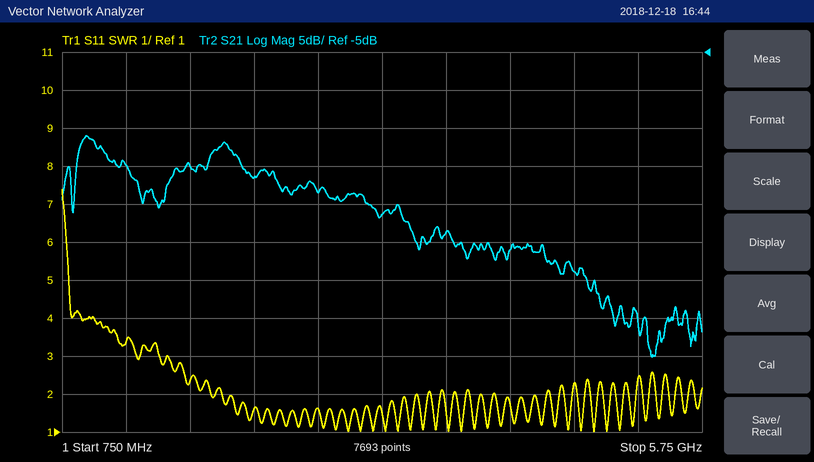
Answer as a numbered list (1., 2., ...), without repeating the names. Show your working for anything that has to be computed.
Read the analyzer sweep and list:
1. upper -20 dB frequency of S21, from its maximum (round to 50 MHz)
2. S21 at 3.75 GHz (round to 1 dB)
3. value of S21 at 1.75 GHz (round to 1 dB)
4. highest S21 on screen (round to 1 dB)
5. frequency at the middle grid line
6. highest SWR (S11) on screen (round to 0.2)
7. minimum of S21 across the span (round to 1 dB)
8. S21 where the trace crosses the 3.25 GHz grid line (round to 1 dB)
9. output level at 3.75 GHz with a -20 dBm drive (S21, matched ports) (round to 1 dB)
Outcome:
1. 4.85 GHz
2. -29 dB
3. -20 dB
4. -16 dB
5. 3.25 GHz
6. 7.4
7. -45 dB
8. -26 dB
9. -20 dBm + (-29 dB) = -49 dBm
